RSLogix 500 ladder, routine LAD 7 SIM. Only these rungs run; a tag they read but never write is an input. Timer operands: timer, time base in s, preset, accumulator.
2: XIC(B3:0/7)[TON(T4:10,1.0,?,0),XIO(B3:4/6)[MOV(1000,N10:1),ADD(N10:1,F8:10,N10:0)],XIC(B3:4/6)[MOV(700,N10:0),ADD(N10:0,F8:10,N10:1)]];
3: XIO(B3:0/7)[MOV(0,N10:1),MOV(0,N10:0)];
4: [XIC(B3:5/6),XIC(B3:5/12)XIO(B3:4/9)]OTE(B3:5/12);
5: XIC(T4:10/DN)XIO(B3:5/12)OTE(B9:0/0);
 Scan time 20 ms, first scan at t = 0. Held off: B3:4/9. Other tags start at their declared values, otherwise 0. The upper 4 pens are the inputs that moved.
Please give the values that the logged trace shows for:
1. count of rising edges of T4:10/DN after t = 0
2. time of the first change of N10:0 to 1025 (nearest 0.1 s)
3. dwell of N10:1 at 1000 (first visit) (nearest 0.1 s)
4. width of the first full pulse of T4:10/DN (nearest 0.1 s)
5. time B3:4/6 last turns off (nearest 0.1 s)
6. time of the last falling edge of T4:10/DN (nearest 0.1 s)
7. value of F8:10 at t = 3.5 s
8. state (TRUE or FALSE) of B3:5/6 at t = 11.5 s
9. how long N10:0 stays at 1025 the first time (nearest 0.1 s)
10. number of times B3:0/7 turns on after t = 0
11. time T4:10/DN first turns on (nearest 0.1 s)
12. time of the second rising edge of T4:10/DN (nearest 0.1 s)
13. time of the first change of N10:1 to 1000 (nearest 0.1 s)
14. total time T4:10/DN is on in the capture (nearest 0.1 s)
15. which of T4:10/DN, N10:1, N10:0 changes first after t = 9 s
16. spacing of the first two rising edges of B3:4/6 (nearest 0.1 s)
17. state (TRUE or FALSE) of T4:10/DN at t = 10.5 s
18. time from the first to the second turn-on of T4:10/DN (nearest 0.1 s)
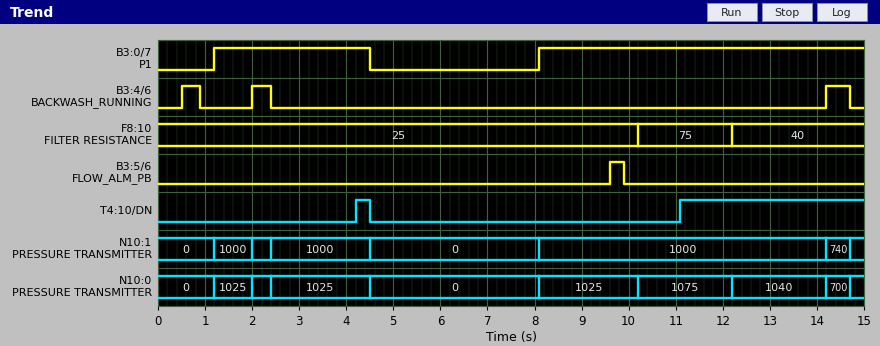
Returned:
2
1.2 s
0.8 s
0.3 s
14.7 s
4.5 s
25
FALSE
0.8 s
2
4.2 s
11.1 s
1.2 s
4.2 s
N10:0
1.5 s
FALSE
6.9 s
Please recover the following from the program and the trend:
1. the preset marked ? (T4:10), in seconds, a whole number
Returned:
3 s
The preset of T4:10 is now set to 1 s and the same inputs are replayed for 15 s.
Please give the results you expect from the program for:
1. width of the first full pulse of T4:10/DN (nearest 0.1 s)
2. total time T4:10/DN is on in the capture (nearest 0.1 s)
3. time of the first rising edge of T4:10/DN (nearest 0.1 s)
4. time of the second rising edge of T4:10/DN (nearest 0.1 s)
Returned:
2.3 s
8.2 s
2.2 s
9.1 s
